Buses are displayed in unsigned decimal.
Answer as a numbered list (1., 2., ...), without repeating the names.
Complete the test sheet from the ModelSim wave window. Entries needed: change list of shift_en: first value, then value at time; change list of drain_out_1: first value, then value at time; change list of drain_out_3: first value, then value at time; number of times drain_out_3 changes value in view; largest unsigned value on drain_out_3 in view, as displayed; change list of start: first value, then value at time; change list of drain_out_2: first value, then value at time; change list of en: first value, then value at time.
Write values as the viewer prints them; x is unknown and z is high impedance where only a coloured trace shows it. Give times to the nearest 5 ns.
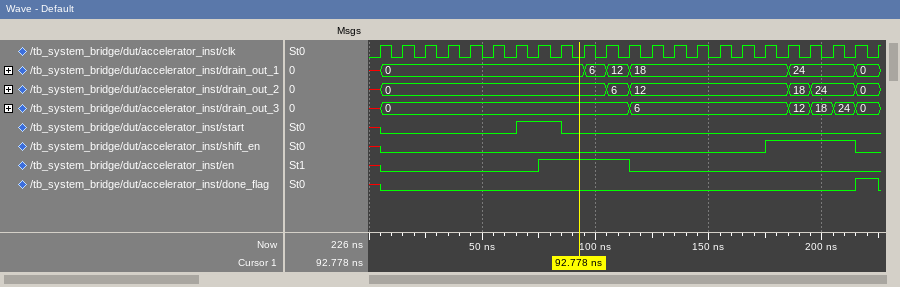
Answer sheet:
1. x, 0 at 5 ns, 1 at 175 ns, 0 at 215 ns
2. x, 0 at 5 ns, 6 at 95 ns, 12 at 105 ns, 18 at 115 ns, 24 at 185 ns, 0 at 215 ns
3. x, 0 at 5 ns, 6 at 115 ns, 12 at 185 ns, 18 at 195 ns, 24 at 205 ns, 0 at 215 ns
4. 6
5. 24
6. x, 0 at 5 ns, 1 at 65 ns, 0 at 85 ns
7. x, 0 at 5 ns, 6 at 105 ns, 12 at 115 ns, 18 at 185 ns, 24 at 195 ns, 0 at 215 ns
8. x, 0 at 5 ns, 1 at 75 ns, 0 at 115 ns
